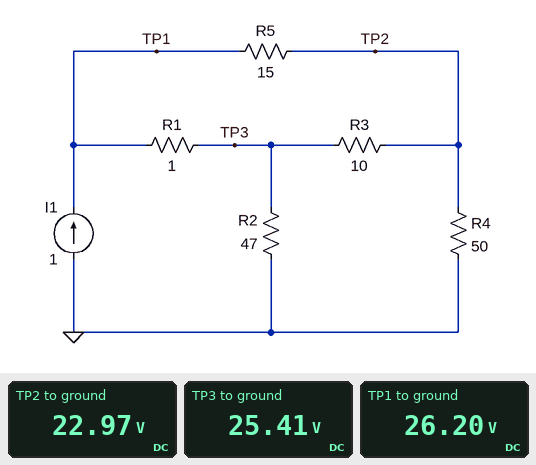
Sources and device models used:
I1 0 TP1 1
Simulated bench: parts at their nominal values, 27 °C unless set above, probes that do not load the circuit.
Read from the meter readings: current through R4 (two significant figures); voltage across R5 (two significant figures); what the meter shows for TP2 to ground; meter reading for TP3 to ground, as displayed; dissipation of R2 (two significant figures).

460 mA
3.2 V
22.97 V
25.41 V
14 W
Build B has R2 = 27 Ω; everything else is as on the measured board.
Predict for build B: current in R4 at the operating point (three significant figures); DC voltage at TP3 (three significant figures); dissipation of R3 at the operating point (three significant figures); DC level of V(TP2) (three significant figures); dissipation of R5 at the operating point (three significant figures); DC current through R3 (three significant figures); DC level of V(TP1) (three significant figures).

329 mA
18.1 V
270 mW
16.5 V
409 mW
164 mA
18.9 V
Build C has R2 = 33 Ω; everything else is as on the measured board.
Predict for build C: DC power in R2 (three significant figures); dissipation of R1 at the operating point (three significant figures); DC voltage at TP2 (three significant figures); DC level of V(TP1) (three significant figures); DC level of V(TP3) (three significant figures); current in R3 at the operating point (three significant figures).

12.9 W
668 mW
18.7 V
21.5 V
20.6 V
192 mA
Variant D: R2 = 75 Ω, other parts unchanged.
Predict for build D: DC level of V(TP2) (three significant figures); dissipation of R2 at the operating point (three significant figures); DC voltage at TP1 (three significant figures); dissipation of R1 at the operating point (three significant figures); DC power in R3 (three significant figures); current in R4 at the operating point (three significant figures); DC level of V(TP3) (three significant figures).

28.7 V
13.6 W
32.6 V
548 mW
994 mW
575 mA
31.9 V
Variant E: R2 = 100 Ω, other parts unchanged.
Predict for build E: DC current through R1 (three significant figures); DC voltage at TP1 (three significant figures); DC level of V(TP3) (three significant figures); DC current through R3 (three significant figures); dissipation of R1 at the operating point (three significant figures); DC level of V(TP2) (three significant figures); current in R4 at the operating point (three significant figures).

714 mA
36.4 V
35.7 V
357 mA
510 mW
32.1 V
643 mA
